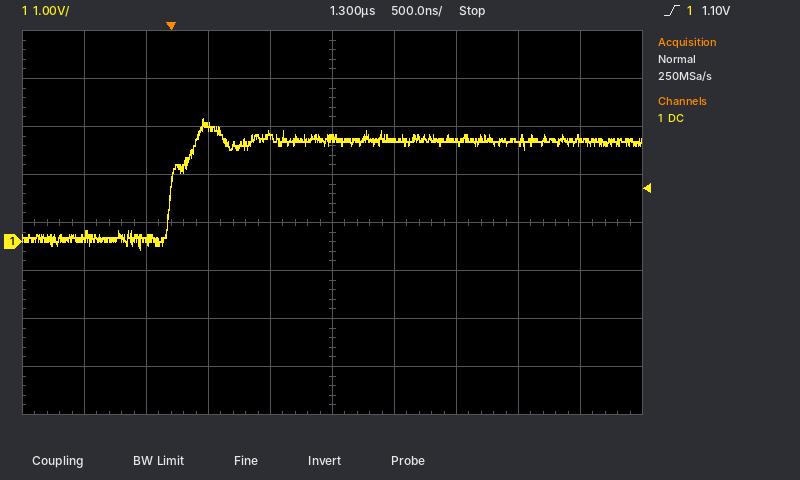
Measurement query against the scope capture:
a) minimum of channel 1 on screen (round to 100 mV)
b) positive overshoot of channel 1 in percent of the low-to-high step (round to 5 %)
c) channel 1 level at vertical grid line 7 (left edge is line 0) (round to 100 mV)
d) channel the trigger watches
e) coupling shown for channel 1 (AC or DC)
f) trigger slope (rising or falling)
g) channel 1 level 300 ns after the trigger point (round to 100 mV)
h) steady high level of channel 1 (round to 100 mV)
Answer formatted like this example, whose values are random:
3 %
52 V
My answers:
-200 mV
20 %
2.1 V
channel 1
DC
rising
2.4 V
2.1 V
